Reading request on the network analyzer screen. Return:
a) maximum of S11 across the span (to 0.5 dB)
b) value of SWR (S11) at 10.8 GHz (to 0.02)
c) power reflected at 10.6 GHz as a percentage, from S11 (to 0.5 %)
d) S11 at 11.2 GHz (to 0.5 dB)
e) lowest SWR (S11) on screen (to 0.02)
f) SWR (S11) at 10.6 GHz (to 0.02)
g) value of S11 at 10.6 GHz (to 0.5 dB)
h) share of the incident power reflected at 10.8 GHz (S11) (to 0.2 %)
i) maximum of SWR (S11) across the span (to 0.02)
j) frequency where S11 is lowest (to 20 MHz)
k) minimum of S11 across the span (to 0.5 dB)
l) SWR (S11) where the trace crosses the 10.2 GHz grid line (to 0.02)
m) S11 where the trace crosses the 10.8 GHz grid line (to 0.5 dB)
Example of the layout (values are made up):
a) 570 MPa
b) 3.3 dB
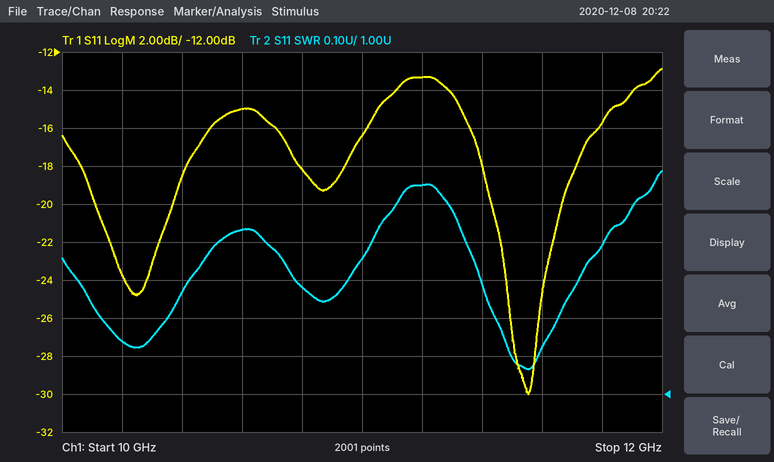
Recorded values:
a) -13.0 dB
b) 1.28
c) 3.0 %
d) -13.5 dB
e) 1.06
f) 1.44
g) -15.0 dB
h) 1.6 %
i) 1.58
j) 11.56 GHz
k) -30.0 dB
l) 1.14
m) -18.0 dB
